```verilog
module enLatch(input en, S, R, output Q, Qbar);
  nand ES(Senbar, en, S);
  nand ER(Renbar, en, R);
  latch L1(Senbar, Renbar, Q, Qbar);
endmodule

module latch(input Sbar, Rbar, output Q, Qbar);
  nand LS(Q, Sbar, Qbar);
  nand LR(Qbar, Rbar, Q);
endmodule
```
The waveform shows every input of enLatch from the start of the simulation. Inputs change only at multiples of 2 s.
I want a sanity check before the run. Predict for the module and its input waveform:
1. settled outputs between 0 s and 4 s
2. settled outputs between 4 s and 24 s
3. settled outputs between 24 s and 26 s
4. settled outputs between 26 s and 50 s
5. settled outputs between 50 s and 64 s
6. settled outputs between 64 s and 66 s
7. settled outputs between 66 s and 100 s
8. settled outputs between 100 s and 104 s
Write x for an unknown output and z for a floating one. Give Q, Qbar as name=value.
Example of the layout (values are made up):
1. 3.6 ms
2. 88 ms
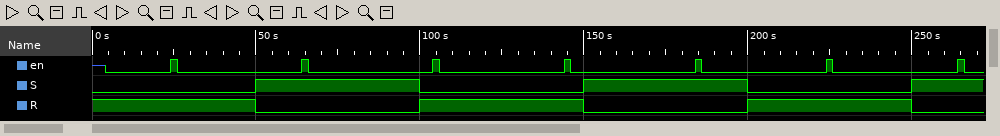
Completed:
1. Q=x, Qbar=x
2. Q=x, Qbar=x
3. Q=0, Qbar=1
4. Q=0, Qbar=1
5. Q=0, Qbar=1
6. Q=1, Qbar=0
7. Q=1, Qbar=0
8. Q=1, Qbar=0
